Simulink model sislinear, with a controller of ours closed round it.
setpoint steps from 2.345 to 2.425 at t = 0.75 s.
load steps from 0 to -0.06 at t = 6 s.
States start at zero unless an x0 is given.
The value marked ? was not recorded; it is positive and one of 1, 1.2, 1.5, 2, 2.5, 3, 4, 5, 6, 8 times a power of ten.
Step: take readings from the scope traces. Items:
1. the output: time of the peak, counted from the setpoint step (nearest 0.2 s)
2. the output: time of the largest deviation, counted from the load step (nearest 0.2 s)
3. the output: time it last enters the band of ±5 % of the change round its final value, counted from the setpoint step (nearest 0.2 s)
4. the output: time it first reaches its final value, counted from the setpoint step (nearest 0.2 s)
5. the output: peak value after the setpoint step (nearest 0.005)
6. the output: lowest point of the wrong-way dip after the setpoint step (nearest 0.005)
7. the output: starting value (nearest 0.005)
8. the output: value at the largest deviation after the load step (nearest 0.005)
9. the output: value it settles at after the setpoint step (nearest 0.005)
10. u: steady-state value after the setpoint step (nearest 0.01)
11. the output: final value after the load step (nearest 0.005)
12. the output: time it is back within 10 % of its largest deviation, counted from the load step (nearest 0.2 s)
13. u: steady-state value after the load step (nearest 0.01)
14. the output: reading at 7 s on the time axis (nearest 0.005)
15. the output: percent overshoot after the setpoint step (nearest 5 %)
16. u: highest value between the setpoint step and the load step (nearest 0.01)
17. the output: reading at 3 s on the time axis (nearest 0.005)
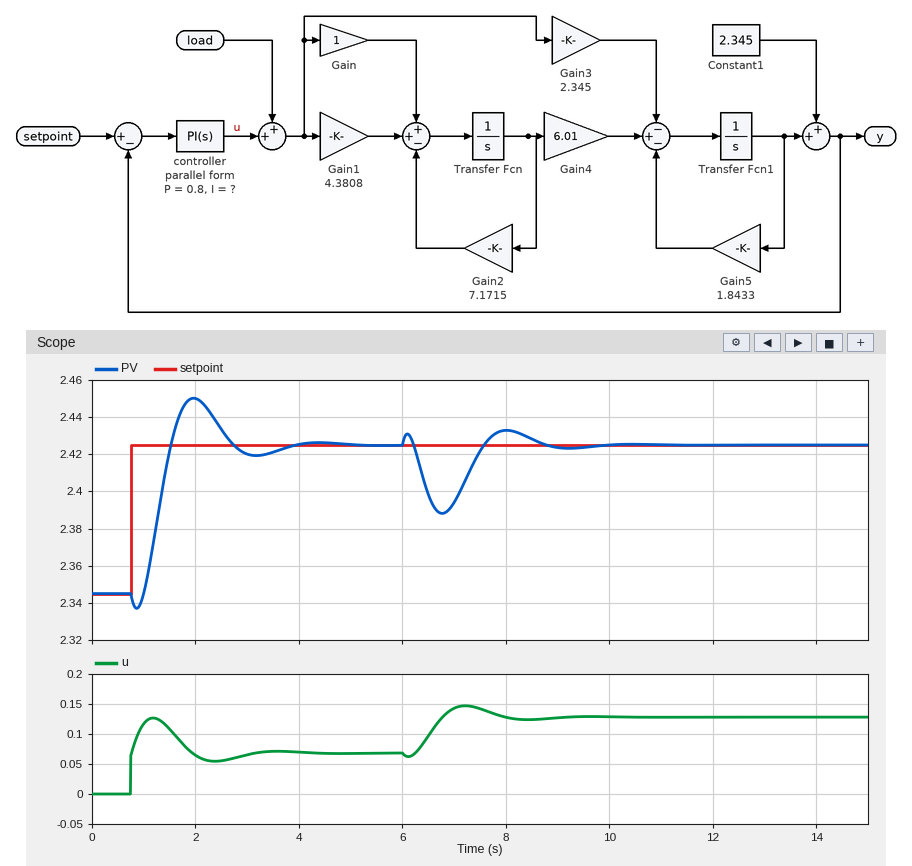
1.2 s
0.8 s
2.8 s
0.8 s
2.450
2.335
2.345
2.390
2.425
0.07
2.425
2.4 s
0.13
2.395
30 %
0.13
2.420
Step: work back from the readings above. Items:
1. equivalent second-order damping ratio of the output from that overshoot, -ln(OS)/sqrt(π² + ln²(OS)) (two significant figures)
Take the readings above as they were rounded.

0.36
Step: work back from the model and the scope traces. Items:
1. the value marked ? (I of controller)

2.5
